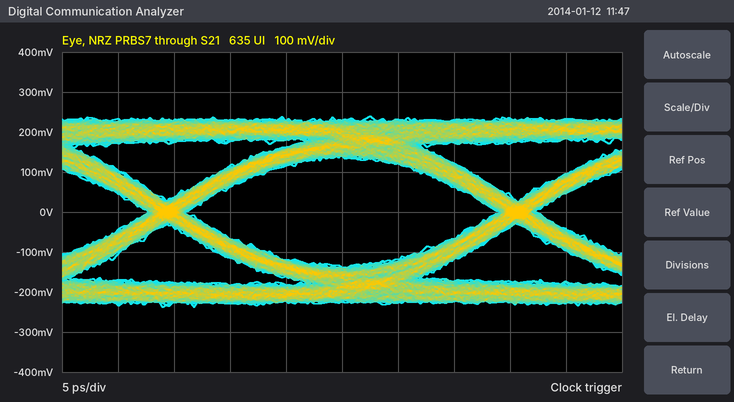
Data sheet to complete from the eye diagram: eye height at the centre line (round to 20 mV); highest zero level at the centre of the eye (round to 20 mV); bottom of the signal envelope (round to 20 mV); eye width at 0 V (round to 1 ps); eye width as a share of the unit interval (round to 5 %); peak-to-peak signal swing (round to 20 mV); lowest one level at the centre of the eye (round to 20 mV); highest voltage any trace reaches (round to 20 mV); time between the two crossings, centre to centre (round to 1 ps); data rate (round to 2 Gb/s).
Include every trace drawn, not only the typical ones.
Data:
280 mV
-140 mV
-240 mV
28 ps
90 %
480 mV
140 mV
240 mV
31 ps
32 Gb/s
